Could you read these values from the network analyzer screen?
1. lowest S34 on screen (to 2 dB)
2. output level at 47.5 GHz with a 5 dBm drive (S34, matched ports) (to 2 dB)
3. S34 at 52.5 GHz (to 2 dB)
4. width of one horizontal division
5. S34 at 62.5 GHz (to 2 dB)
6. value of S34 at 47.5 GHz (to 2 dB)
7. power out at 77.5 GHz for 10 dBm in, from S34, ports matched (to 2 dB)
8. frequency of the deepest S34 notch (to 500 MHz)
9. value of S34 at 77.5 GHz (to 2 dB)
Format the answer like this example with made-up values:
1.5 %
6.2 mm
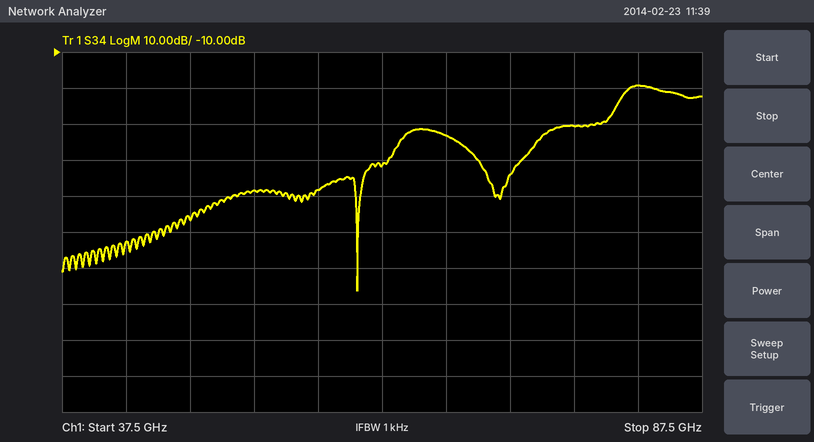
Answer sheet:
-76 dB
-52 dBm
-48 dB
5 GHz
-42 dB
-56 dB
-20 dBm
60.5 GHz
-30 dB
